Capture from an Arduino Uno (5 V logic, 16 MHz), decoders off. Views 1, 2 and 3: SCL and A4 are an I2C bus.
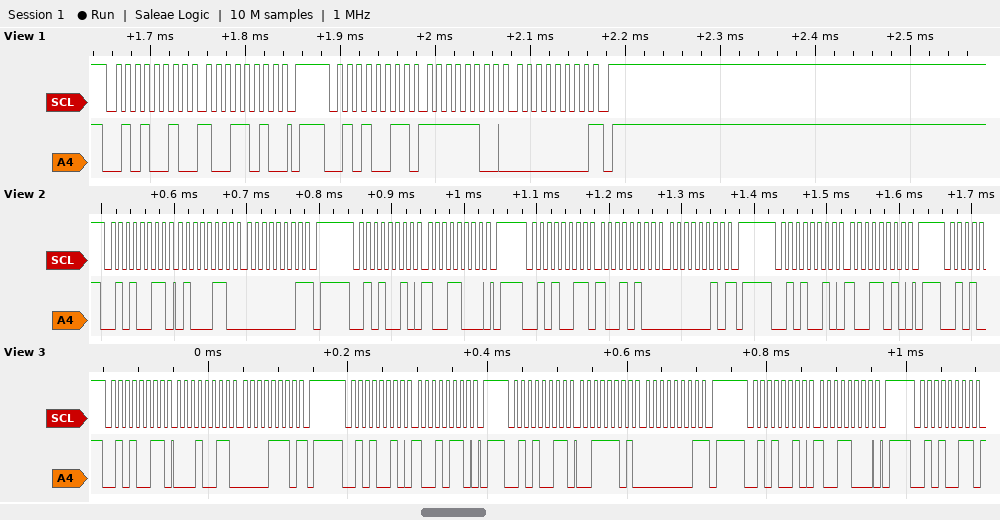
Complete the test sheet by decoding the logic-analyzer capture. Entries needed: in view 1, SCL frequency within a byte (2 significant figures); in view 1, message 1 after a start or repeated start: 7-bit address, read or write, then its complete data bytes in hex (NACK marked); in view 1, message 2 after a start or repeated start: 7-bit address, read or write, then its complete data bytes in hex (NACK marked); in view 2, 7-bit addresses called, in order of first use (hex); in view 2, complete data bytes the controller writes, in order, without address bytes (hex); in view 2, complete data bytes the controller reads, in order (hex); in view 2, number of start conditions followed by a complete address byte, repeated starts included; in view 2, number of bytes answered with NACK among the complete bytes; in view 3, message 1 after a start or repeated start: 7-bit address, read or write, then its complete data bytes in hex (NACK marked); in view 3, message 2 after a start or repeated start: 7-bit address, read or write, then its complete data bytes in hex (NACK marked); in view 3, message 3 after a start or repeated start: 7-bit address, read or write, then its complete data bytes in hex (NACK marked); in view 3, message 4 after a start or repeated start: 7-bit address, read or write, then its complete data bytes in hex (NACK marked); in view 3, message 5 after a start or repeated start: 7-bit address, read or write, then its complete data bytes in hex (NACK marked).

100 kHz
0x29 write: 9A
0x29 read: FC 00 NACK
0x29
98 9A
46 01 94 02
4
2
0x29 read: 13 0E NACK
0x29 write: 96
0x29 read: 3D 01 NACK
0x29 write: 98
0x29 read
